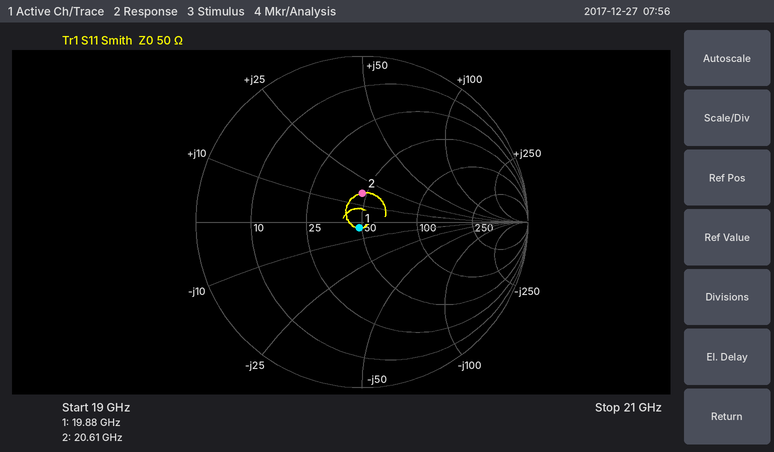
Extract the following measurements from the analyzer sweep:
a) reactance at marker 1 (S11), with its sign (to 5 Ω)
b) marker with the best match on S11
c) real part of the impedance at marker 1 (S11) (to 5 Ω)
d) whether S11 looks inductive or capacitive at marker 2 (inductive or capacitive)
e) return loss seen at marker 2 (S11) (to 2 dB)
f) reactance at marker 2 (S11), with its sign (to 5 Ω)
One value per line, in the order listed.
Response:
-5 Ω
marker 1
50 Ω
inductive
16 dB
+15 Ω
